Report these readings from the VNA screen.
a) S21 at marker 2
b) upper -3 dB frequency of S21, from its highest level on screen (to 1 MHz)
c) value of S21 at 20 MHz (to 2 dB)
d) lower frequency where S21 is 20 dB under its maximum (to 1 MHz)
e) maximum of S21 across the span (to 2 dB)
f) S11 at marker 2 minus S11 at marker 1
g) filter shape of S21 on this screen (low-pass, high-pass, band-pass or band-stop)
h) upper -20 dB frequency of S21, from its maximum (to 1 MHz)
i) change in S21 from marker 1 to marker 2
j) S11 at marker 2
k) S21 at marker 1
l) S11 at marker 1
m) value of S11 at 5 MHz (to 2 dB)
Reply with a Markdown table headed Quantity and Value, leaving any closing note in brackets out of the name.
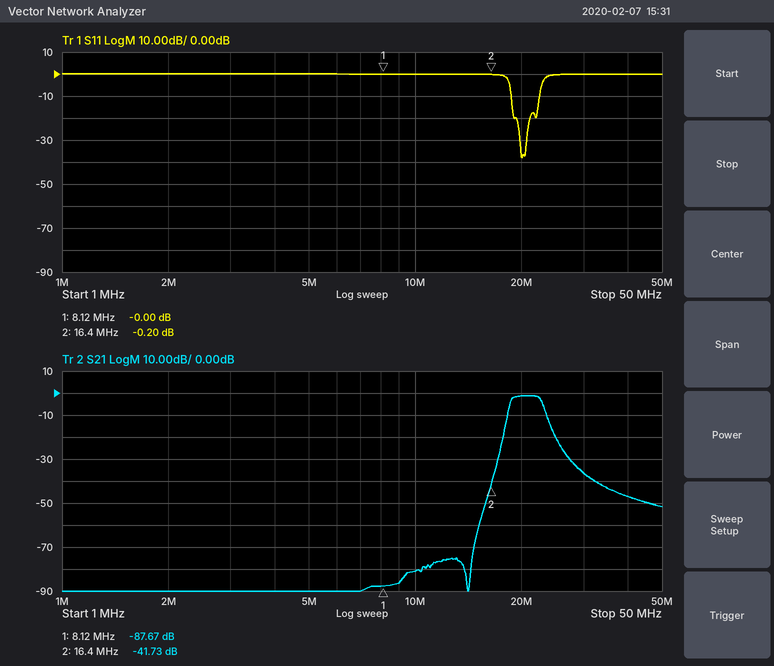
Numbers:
| Quantity | Value |
|---|---|
| S21 at marker 2 | -41.73 dB |
| upper -3 dB frequency of S21, from its highest level on screen | 23 MHz |
| value of S21 at 20 MHz | -2 dB |
| lower frequency where S21 is 20 dB under its maximum | 18 MHz |
| maximum of S21 across the span | -2 dB |
| S11 at marker 2 minus S11 at marker 1 | -0.20 dB |
| filter shape of S21 on this screen | band-pass |
| upper -20 dB frequency of S21, from its maximum | 25 MHz |
| change in S21 from marker 1 to marker 2 | 45.94 dB |
| S11 at marker 2 | -0.20 dB |
| S21 at marker 1 | -87.67 dB |
| S11 at marker 1 | -0.00 dB |
| value of S11 at 5 MHz | 0 dB |
